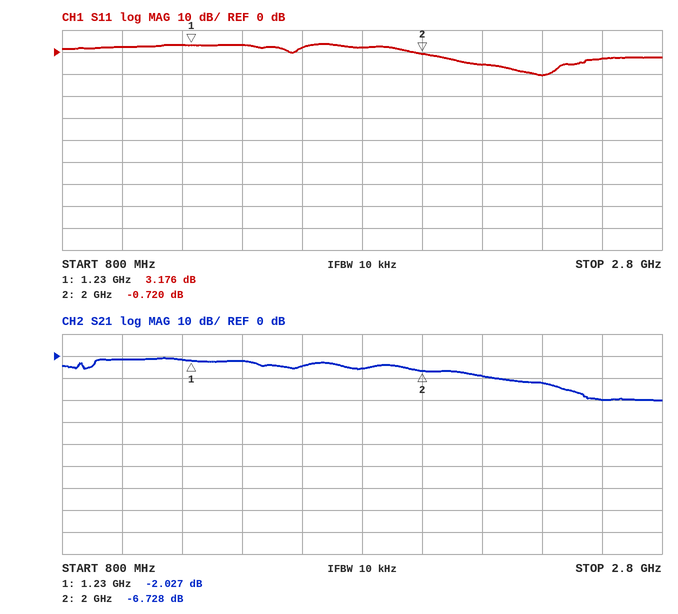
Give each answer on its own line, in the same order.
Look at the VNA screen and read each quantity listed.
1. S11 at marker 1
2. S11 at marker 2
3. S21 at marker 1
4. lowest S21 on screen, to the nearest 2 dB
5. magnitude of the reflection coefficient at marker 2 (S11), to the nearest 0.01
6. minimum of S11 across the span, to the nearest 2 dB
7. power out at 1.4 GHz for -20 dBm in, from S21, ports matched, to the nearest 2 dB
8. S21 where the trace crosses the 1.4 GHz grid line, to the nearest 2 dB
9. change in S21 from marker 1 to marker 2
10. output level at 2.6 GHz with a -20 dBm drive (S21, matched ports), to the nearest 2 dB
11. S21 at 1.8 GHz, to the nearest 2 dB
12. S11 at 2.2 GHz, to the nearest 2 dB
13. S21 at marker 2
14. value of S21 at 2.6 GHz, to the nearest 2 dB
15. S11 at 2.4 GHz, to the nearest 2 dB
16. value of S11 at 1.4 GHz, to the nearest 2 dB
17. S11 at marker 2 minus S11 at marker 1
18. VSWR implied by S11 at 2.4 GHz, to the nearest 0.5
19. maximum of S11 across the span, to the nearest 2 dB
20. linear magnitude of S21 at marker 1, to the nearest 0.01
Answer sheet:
3.176 dB
-0.720 dB
-2.027 dB
-20 dB
0.92
-10 dB
-22 dBm
-2 dB
-4.701 dB
-40 dBm
-6 dB
-6 dB
-6.728 dB
-20 dB
-10 dB
4 dB
-3.896 dB
2.0
4 dB
0.79
